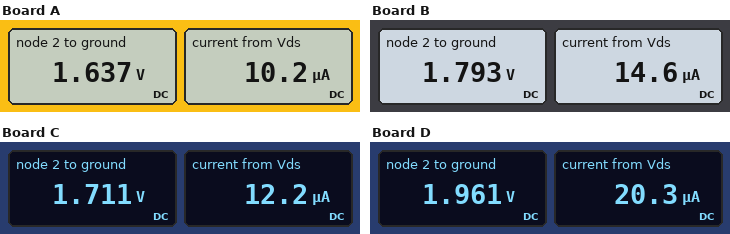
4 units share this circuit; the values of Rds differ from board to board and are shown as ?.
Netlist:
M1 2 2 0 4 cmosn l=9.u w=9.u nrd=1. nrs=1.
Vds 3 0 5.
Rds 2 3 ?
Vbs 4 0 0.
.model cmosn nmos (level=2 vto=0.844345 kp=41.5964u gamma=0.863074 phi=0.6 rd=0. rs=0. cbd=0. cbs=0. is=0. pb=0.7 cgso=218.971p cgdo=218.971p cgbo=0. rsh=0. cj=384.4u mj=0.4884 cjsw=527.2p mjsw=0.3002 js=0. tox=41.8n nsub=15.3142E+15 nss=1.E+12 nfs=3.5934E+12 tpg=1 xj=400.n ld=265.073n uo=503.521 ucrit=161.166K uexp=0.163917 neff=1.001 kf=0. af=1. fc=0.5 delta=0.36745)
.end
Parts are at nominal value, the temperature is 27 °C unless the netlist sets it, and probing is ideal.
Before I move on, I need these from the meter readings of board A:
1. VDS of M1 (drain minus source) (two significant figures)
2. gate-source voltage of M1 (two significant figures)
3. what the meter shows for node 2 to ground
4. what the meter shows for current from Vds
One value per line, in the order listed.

1.6 V
1.6 V
1.637 V
10.2 µA
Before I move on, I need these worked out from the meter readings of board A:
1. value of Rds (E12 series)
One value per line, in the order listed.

330 kΩ
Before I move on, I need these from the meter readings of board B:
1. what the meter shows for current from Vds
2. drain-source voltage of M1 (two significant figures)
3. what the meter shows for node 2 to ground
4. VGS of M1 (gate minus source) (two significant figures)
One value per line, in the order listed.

14.6 µA
1.8 V
1.793 V
1.8 V
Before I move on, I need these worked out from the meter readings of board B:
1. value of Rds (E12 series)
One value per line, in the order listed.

220 kΩ
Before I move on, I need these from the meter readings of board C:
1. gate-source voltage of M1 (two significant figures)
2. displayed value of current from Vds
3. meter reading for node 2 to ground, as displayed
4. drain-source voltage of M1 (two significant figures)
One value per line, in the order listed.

1.7 V
12.2 µA
1.711 V
1.7 V
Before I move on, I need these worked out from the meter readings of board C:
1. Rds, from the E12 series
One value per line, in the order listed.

270 kΩ
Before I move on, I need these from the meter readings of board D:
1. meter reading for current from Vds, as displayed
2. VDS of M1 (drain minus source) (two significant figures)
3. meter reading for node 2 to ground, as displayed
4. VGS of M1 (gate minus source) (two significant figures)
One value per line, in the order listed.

20.3 µA
2.0 V
1.961 V
2.0 V
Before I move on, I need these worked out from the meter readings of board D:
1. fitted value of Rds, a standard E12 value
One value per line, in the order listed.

150 kΩ
